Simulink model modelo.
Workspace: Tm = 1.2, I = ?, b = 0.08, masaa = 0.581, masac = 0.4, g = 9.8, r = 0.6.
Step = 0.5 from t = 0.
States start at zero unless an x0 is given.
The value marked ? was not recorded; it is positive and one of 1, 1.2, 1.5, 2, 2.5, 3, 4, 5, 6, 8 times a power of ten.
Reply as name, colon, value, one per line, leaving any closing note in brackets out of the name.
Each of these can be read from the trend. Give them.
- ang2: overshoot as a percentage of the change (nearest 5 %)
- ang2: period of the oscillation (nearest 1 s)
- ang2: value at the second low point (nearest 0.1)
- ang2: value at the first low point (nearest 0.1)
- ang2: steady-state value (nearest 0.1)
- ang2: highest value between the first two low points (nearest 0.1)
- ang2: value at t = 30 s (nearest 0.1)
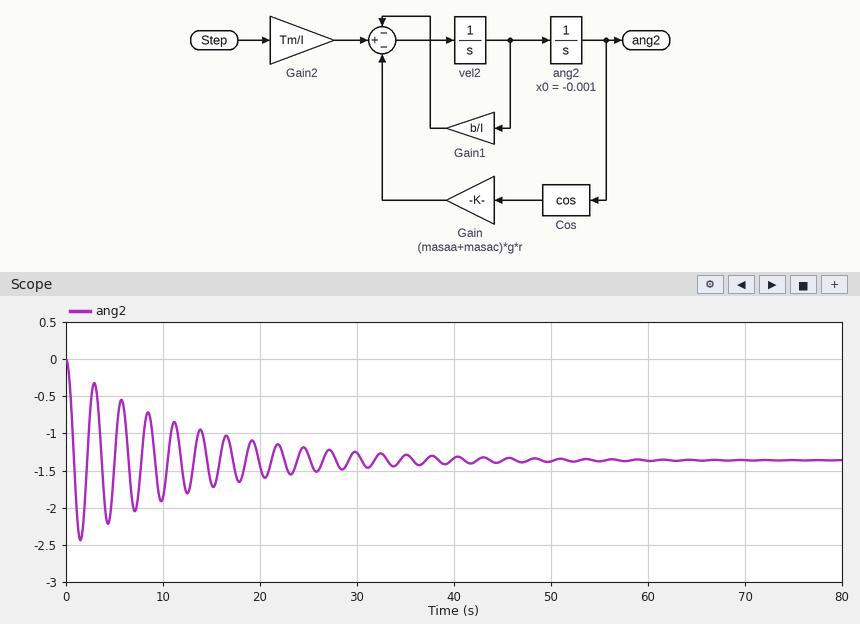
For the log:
ang2: overshoot as a percentage of the change: 80 %
ang2: period of the oscillation: 3 s
ang2: value at the second low point: -2.2
ang2: value at the first low point: -2.4
ang2: steady-state value: -1.4
ang2: highest value between the first two low points: -0.3
ang2: value at t = 30 s: -1.3
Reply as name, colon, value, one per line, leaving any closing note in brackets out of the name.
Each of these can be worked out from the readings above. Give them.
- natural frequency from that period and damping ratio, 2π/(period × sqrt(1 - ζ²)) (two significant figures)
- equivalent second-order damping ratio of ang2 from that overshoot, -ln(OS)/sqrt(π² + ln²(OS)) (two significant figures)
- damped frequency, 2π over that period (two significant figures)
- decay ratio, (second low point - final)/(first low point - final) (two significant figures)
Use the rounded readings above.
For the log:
natural frequency from that period and damping ratio, 2π/(period × sqrt(1 - ζ²)): 2.1 rad/s
equivalent second-order damping ratio of ang2 from that overshoot, -ln(OS)/sqrt(π² + ln²(OS)): 0.071
damped frequency, 2π over that period: 2.1 rad/s
decay ratio, (second low point - final)/(first low point - final): 0.80
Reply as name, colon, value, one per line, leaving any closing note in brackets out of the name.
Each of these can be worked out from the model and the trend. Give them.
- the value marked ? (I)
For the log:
the value marked ?: 0.5
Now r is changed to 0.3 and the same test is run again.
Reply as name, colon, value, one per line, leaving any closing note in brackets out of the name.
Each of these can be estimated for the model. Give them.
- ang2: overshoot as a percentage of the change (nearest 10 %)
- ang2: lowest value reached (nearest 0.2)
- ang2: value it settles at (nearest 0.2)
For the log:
ang2: overshoot as a percentage of the change: 70 %
ang2: lowest value reached: -2.0
ang2: value it settles at: -1.2
